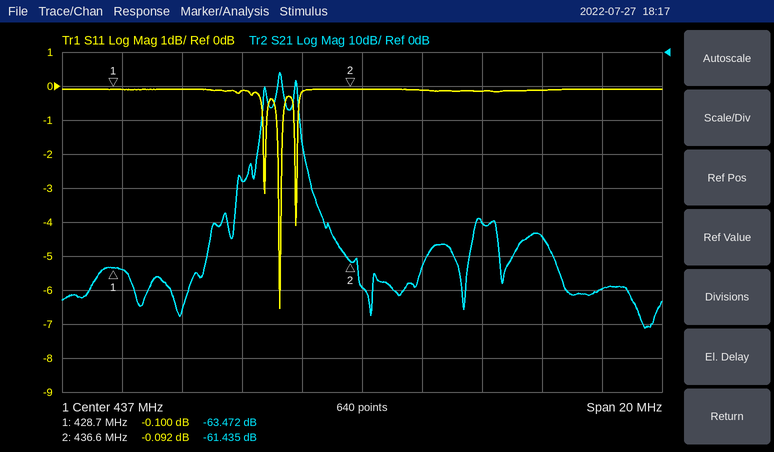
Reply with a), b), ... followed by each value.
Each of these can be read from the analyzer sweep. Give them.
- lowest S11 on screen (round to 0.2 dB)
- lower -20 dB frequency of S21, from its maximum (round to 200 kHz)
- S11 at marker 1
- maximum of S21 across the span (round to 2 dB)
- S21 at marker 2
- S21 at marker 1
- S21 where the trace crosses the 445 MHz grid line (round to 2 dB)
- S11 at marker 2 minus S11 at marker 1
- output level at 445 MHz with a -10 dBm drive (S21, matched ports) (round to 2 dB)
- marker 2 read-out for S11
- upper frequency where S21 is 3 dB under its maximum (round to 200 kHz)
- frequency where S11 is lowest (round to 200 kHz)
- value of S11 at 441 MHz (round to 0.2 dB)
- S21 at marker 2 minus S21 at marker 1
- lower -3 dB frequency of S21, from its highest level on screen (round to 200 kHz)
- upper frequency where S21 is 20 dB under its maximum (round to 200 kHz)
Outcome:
a) -6.6 dB
b) 433.6 MHz
c) -0.100 dB
d) -6 dB
e) -61.435 dB
f) -63.472 dB
g) -70 dB
h) 0.008 dB
i) -80 dBm
j) -0.092 dB
k) 434.4 MHz
l) 434.2 MHz
m) -0.2 dB
n) 2.037 dB
o) 434.2 MHz
p) 435.0 MHz
